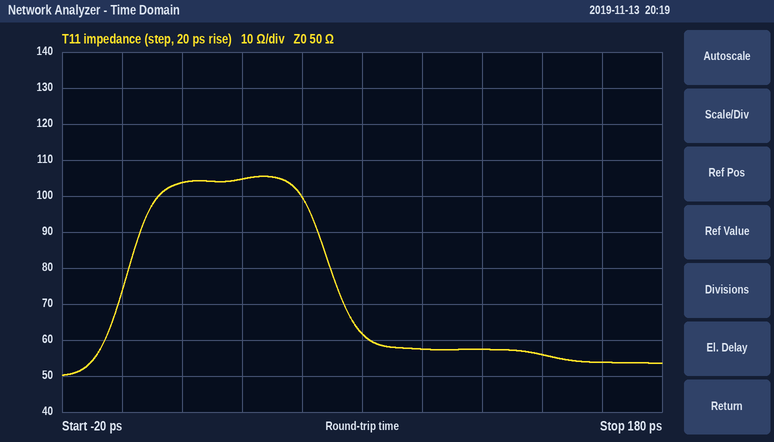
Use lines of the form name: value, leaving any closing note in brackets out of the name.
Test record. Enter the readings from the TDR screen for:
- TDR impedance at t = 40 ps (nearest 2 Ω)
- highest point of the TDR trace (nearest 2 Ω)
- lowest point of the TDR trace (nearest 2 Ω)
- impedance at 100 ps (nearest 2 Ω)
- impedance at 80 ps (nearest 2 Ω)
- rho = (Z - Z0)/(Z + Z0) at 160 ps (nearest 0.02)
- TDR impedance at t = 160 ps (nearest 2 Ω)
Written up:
TDR impedance at t = 40 ps: 104 Ω
highest point of the TDR trace: 106 Ω
lowest point of the TDR trace: 50 Ω
impedance at 100 ps: 58 Ω
impedance at 80 ps: 62 Ω
rho = (Z - Z0)/(Z + Z0) at 160 ps: +0.04
TDR impedance at t = 160 ps: 54 Ω
